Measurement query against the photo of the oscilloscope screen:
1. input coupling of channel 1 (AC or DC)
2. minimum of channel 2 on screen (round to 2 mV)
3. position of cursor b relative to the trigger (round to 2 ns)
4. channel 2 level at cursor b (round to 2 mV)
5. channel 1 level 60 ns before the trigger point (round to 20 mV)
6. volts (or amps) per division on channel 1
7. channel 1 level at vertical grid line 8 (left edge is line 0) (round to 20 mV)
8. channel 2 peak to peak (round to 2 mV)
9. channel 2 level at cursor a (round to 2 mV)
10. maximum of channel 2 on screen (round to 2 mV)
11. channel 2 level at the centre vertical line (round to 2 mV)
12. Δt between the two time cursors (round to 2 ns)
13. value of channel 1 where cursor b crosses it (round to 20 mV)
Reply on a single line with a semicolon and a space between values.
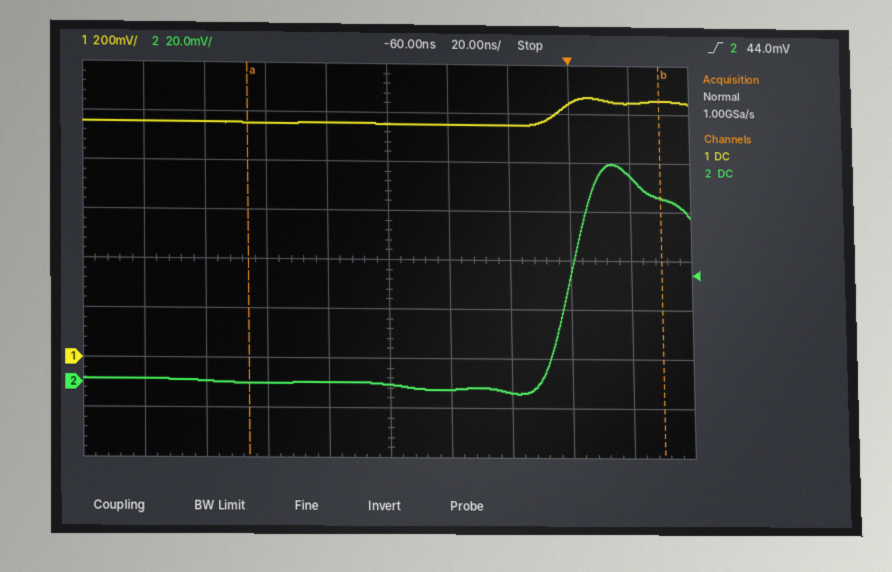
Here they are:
DC; -4 mV; +30 ns; 76 mV; 960 mV; 200 mV; 1.04 V; 94 mV; 0 mV; 90 mV; 0 mV; 136 ns; 1.06 V
